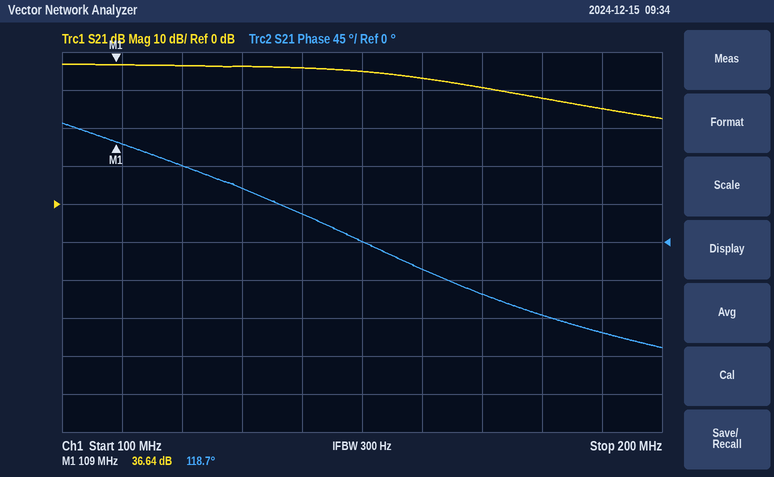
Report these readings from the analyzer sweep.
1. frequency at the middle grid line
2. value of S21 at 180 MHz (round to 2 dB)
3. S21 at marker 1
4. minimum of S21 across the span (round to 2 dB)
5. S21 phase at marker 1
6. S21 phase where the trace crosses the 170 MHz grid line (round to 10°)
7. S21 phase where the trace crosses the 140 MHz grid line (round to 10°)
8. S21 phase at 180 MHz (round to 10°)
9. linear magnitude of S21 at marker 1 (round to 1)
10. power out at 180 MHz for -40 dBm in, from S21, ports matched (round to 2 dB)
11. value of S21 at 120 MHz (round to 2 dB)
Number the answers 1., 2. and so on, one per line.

1. 150 MHz
2. 28 dB
3. 36.64 dB
4. 22 dB
5. 118.7°
6. -60°
7. 30°
8. -90°
9. 68
10. -12 dBm
11. 36 dB
